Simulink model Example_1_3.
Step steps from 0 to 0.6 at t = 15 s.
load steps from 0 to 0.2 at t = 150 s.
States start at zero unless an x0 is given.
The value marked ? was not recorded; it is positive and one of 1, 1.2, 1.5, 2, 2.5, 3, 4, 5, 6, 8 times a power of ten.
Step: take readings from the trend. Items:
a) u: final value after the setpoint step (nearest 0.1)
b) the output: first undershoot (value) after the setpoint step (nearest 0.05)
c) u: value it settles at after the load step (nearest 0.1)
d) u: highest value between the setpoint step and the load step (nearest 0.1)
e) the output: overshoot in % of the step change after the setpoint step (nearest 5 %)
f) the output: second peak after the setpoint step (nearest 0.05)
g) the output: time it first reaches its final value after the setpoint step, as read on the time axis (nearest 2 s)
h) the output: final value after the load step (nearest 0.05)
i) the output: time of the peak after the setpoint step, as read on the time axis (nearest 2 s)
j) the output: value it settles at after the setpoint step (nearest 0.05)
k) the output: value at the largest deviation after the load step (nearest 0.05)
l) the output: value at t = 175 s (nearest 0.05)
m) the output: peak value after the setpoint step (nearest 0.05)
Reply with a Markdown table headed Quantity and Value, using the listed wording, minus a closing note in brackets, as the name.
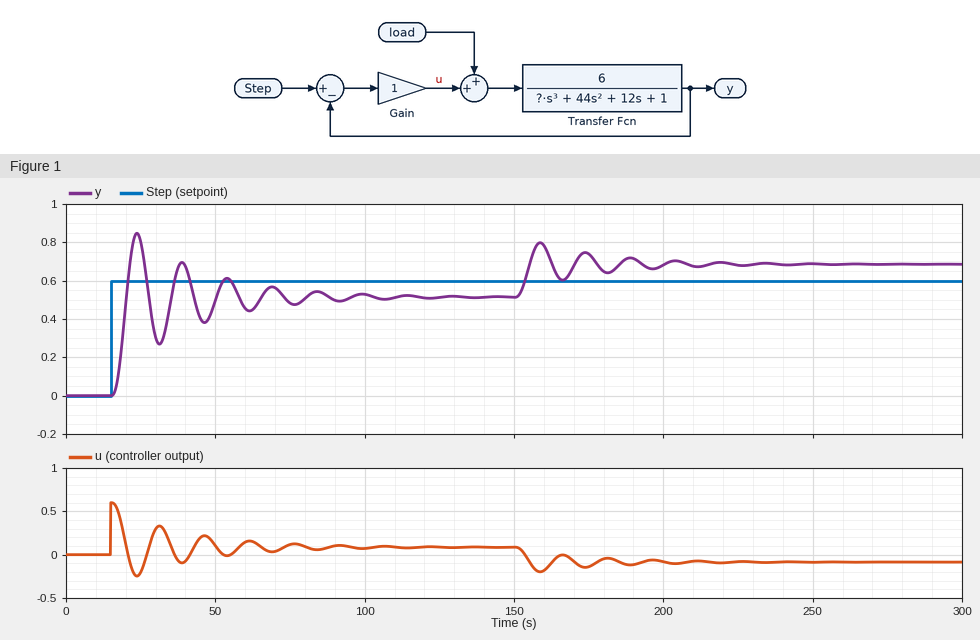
| Quantity | Value |
|---|---|
| u: final value after the setpoint step | 0.1 |
| the output: first undershoot (value) after the setpoint step | 0.25 |
| u: value it settles at after the load step | -0.1 |
| u: highest value between the setpoint step and the load step | 0.6 |
| the output: overshoot in % of the step change after the setpoint step | 65 % |
| the output: second peak after the setpoint step | 0.70 |
| the output: time it first reaches its final value after the setpoint step, as read on the time axis | 20 s |
| the output: final value after the load step | 0.70 |
| the output: time of the peak after the setpoint step, as read on the time axis | 24 s |
| the output: value it settles at after the setpoint step | 0.50 |
| the output: value at the largest deviation after the load step | 0.80 |
| the output: value at t = 175 s | 0.75 |
| the output: peak value after the setpoint step | 0.85 |
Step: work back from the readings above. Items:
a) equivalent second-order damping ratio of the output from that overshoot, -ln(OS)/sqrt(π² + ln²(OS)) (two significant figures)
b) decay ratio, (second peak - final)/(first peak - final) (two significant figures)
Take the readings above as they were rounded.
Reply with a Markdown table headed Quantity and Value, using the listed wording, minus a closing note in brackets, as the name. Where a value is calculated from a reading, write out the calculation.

| Quantity | Value |
|---|---|
| equivalent second-order damping ratio of the output from that overshoot, -ln(OS)/sqrt(π² + ln²(OS)) | ln(0.65) = -0.431; 0.431 / sqrt(9.870 + 0.186) = 0.14 |
| decay ratio, (second peak - final)/(first peak - final) | (0.7 - 0.5) / (0.85 - 0.5) = 0.57 |
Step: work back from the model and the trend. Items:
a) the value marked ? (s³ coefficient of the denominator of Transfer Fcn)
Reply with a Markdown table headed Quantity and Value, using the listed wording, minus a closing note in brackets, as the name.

| Quantity | Value |
|---|---|
| the value marked ? | 50 |
